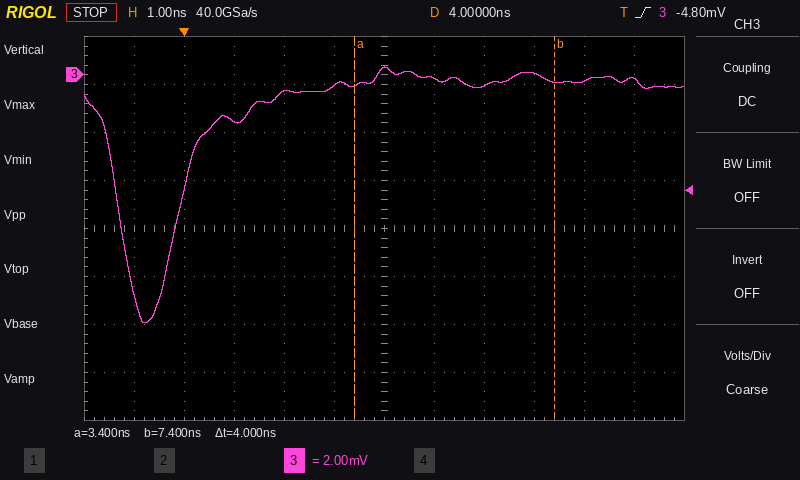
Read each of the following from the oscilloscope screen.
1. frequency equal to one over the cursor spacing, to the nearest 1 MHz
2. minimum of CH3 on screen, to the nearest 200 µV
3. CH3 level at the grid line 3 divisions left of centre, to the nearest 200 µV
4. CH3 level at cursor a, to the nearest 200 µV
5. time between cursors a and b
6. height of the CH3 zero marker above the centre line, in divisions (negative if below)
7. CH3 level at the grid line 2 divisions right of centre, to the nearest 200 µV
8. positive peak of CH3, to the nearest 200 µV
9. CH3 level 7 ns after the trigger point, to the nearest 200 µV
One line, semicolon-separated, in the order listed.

250 MHz; -10.4 mV; -2.0 mV; -400 µV; 4 ns; +3.2 div; -400 µV; 400 µV; 0.0 mV
